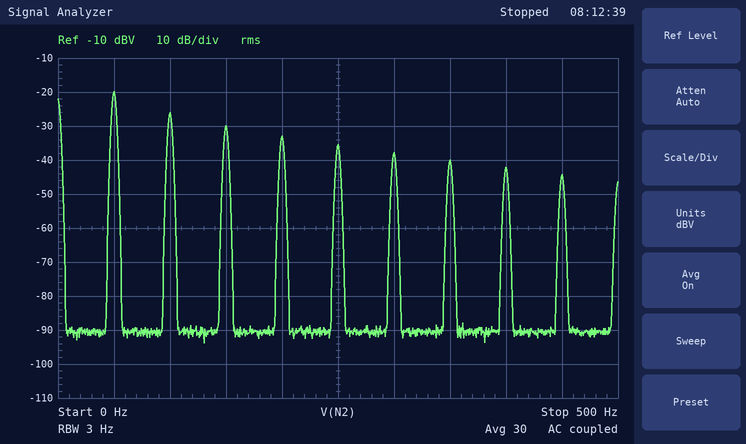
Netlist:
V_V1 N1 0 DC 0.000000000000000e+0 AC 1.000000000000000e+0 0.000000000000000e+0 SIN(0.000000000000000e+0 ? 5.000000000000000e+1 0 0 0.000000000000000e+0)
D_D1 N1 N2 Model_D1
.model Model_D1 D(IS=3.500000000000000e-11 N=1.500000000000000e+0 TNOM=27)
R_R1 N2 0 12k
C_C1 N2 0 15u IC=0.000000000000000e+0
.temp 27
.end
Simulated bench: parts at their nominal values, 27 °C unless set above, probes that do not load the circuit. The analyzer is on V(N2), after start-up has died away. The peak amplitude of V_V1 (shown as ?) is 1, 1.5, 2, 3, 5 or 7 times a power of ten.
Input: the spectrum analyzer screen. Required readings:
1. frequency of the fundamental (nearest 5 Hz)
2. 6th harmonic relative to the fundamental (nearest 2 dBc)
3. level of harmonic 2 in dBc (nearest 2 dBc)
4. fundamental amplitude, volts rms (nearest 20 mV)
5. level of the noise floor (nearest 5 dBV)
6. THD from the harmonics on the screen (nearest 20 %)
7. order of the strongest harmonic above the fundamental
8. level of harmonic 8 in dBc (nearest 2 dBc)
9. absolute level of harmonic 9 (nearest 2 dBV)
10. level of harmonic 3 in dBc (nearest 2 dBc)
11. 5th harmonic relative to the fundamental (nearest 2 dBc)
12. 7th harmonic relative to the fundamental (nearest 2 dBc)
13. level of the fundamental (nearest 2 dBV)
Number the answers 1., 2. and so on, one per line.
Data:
1. 50 Hz
2. -18 dBc
3. -6 dBc
4. 100 mV
5. -90 dBV
6. 60 %
7. 2
8. -22 dBc
9. -44 dBV
10. -10 dBc
11. -16 dBc
12. -20 dBc
13. -20 dBV
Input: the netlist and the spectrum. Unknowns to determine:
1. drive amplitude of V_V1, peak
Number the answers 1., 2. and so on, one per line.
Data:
1. 5 V
